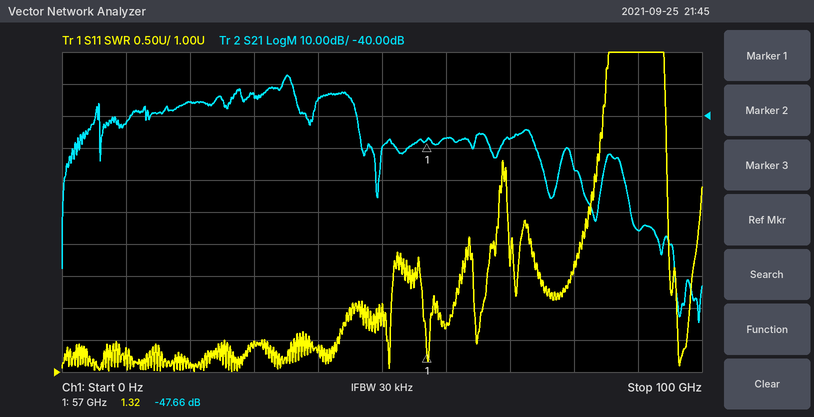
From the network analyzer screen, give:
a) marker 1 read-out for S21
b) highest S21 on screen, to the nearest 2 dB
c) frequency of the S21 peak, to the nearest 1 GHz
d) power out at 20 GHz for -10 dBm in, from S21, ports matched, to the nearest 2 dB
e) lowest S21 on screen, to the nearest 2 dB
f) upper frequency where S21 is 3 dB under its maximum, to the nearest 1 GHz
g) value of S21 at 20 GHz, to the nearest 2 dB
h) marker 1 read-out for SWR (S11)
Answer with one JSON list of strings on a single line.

["-47.66 dB", "-28 dB", "35 GHz", "-46 dBm", "-104 dB", "36 GHz", "-36 dB", "1.32"]
